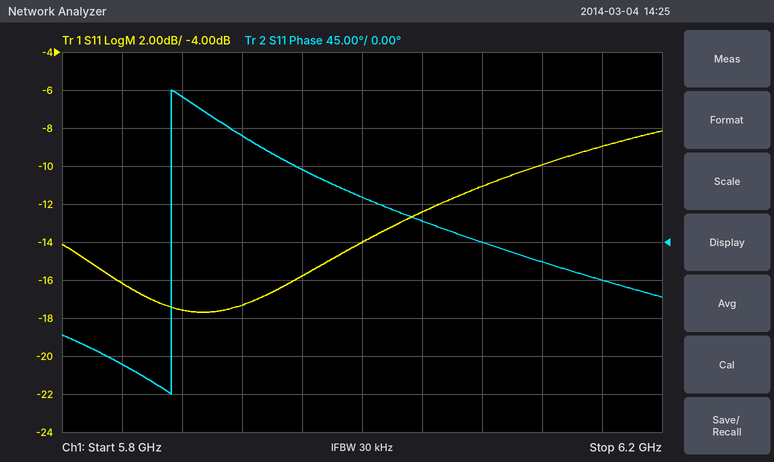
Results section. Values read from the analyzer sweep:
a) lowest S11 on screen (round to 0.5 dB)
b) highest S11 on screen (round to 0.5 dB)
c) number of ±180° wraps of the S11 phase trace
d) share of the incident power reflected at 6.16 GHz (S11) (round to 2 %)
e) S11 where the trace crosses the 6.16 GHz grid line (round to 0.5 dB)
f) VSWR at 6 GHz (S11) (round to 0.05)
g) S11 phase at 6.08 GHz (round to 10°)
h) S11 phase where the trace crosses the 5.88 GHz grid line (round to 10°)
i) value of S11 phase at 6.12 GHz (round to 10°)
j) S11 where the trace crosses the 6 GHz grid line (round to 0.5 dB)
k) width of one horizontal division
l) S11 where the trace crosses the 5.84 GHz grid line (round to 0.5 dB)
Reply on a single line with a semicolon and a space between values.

-17.5 dB; -8.0 dB; 1; 12 %; -9.0 dB; 1.50; 0°; 170°; -20°; -14.0 dB; 40 MHz; -16.0 dB
